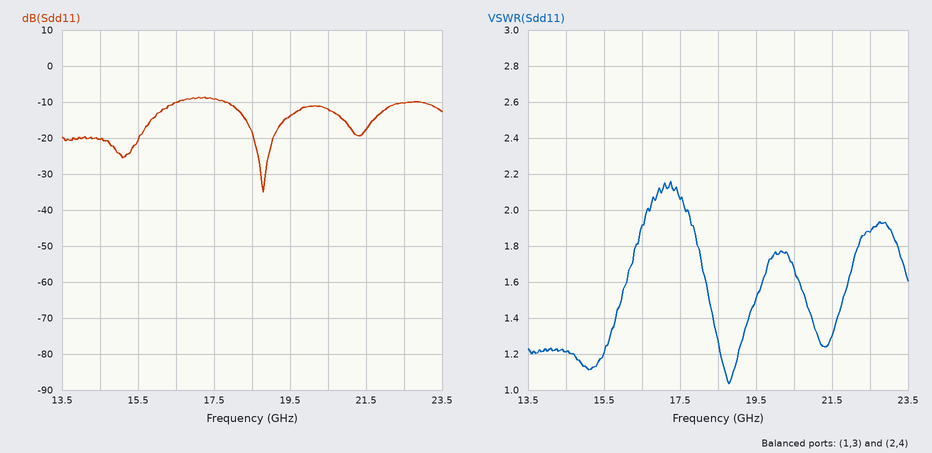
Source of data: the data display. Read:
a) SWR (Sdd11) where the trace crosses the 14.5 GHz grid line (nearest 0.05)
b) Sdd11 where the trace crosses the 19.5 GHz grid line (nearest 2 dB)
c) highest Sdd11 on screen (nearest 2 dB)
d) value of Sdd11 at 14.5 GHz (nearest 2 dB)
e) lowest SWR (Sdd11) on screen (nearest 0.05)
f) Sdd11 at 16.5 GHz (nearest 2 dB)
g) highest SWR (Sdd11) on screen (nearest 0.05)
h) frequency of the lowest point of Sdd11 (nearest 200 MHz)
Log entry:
1.20
-14 dB
-8 dB
-20 dB
1.05
-10 dB
2.15
18.8 GHz
